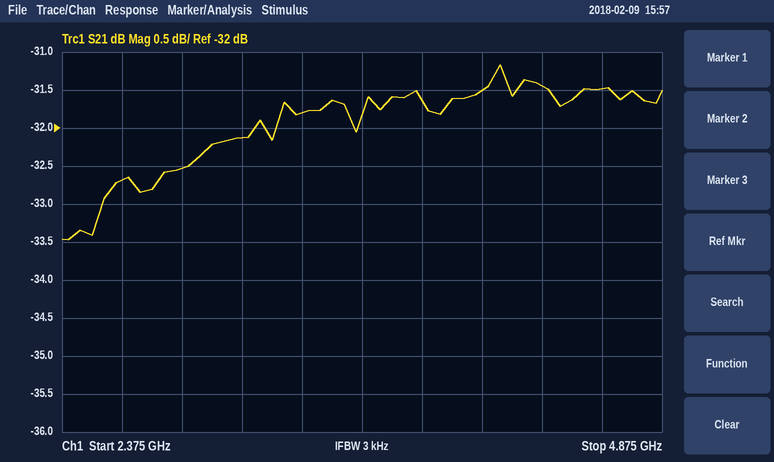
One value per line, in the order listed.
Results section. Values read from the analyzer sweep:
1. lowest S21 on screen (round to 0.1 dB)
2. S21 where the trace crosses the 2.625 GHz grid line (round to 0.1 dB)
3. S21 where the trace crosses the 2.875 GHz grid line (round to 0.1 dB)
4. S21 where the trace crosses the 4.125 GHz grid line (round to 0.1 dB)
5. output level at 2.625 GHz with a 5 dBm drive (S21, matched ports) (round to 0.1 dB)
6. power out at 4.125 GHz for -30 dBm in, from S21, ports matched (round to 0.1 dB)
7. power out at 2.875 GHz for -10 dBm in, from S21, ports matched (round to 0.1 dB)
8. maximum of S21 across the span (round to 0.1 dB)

-33.5 dB
-32.7 dB
-32.5 dB
-31.5 dB
-27.7 dBm
-61.5 dBm
-42.5 dBm
-31.2 dB
